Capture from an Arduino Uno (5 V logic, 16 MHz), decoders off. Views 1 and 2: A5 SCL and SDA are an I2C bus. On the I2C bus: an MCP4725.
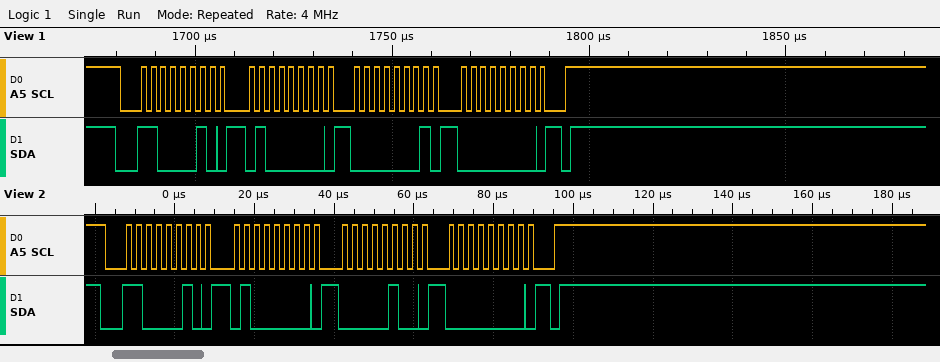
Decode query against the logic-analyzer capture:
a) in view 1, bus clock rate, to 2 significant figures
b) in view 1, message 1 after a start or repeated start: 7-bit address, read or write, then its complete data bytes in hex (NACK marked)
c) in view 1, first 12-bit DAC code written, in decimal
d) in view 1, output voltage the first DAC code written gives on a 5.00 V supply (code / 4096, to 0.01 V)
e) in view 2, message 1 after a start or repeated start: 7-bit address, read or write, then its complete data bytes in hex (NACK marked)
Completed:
400 kHz
0x61 write: 40 01 00
16
0.02 V
0x61 write: 40 04 00
